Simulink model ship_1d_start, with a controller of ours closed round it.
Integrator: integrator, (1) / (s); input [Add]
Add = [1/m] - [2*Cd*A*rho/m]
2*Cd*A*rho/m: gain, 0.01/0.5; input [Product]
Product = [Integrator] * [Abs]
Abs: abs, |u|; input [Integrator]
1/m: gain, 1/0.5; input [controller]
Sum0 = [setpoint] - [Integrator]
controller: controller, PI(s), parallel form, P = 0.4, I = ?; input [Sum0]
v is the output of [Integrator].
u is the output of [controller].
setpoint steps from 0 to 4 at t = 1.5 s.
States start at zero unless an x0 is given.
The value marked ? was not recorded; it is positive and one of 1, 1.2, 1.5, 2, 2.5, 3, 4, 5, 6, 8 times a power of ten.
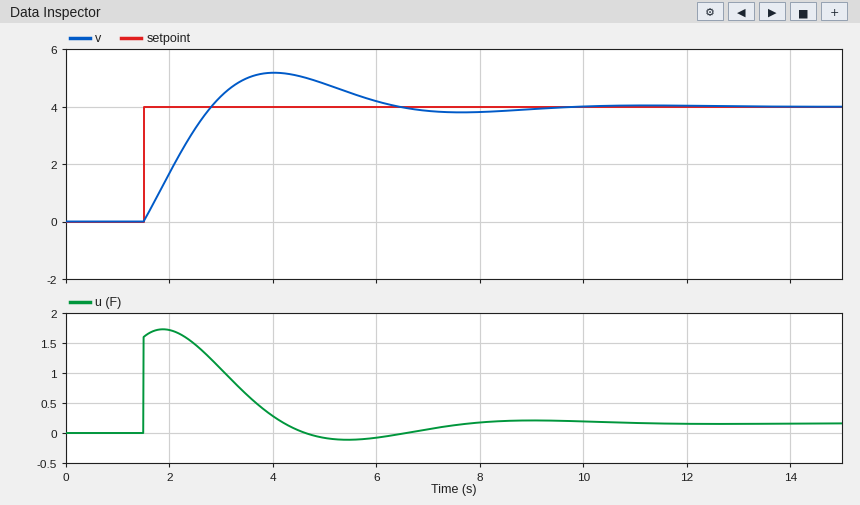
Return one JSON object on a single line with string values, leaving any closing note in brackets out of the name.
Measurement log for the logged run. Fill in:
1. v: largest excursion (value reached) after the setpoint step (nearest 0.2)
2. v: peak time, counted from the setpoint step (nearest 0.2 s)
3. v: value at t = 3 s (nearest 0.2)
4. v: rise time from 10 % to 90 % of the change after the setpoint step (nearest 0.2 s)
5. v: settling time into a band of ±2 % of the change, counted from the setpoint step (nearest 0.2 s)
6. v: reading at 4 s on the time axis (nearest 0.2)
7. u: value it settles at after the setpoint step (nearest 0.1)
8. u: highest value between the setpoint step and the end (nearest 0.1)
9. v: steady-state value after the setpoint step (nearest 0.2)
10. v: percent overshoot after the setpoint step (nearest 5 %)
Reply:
{"v: largest excursion (value reached) after the setpoint step": "5.2", "v: peak time, counted from the setpoint step": "2.6 s", "v: value at t = 3 s": "4.4", "v: rise time from 10 % to 90 % of the change after the setpoint step": "1.0 s", "v: settling time into a band of ±2 % of the change, counted from the setpoint step": "7.6 s", "v: reading at 4 s on the time axis": "5.2", "u: value it settles at after the setpoint step": "0.2", "u: highest value between the setpoint step and the end": "1.7", "v: steady-state value after the setpoint step": "4.0", "v: percent overshoot after the setpoint step": "30 %"}
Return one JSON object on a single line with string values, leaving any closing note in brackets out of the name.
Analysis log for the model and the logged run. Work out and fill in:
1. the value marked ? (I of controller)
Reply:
{"the value marked ?": "0.5"}
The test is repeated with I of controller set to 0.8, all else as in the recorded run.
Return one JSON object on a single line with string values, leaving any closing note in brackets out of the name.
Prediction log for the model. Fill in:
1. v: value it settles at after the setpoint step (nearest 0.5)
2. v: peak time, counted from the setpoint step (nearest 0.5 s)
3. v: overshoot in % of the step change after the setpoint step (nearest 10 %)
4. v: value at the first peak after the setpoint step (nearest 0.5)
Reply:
{"v: value it settles at after the setpoint step": "4.0", "v: peak time, counted from the setpoint step": "2.0 s", "v: overshoot in % of the step change after the setpoint step": "40 %", "v: value at the first peak after the setpoint step": "5.5"}
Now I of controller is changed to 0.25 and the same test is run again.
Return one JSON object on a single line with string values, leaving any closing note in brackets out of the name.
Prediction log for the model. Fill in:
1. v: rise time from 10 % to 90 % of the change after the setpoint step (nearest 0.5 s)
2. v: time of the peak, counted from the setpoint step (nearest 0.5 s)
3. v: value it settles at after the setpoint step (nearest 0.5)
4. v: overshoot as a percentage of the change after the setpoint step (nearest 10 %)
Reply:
{"v: rise time from 10 % to 90 % of the change after the setpoint step": "1.5 s", "v: time of the peak, counted from the setpoint step": "3.5 s", "v: value it settles at after the setpoint step": "4.0", "v: overshoot as a percentage of the change after the setpoint step": "20 %"}
